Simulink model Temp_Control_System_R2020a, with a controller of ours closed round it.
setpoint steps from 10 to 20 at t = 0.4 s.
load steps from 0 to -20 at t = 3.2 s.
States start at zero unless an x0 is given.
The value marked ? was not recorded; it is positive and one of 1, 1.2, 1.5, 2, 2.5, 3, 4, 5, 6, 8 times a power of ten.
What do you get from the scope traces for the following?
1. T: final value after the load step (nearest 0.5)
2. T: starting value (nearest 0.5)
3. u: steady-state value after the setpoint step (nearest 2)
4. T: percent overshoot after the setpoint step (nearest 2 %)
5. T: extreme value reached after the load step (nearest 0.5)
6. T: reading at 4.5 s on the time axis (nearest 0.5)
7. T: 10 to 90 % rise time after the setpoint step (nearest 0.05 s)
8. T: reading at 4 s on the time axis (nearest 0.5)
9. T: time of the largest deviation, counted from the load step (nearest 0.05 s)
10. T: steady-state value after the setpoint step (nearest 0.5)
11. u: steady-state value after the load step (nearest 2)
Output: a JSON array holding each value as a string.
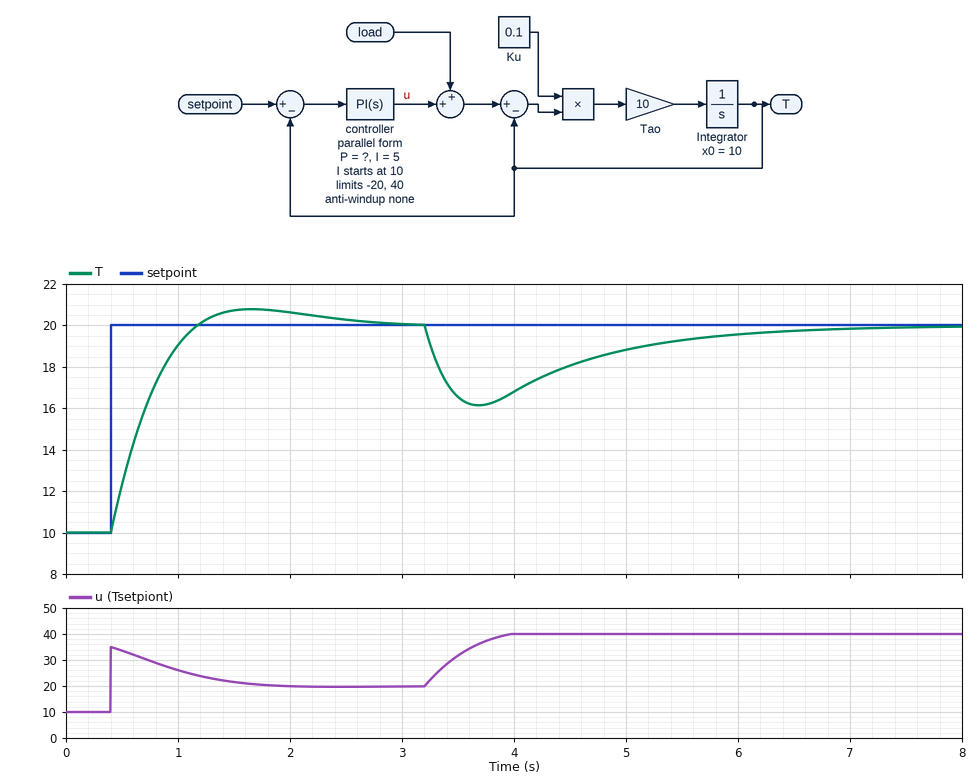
["20.0", "10.0", "20", "8 %", "16.0", "18.0", "0.55 s", "17.0", "0.50 s", "20.0", "40"]
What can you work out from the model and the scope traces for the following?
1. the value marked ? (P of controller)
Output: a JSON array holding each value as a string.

["2.5"]
